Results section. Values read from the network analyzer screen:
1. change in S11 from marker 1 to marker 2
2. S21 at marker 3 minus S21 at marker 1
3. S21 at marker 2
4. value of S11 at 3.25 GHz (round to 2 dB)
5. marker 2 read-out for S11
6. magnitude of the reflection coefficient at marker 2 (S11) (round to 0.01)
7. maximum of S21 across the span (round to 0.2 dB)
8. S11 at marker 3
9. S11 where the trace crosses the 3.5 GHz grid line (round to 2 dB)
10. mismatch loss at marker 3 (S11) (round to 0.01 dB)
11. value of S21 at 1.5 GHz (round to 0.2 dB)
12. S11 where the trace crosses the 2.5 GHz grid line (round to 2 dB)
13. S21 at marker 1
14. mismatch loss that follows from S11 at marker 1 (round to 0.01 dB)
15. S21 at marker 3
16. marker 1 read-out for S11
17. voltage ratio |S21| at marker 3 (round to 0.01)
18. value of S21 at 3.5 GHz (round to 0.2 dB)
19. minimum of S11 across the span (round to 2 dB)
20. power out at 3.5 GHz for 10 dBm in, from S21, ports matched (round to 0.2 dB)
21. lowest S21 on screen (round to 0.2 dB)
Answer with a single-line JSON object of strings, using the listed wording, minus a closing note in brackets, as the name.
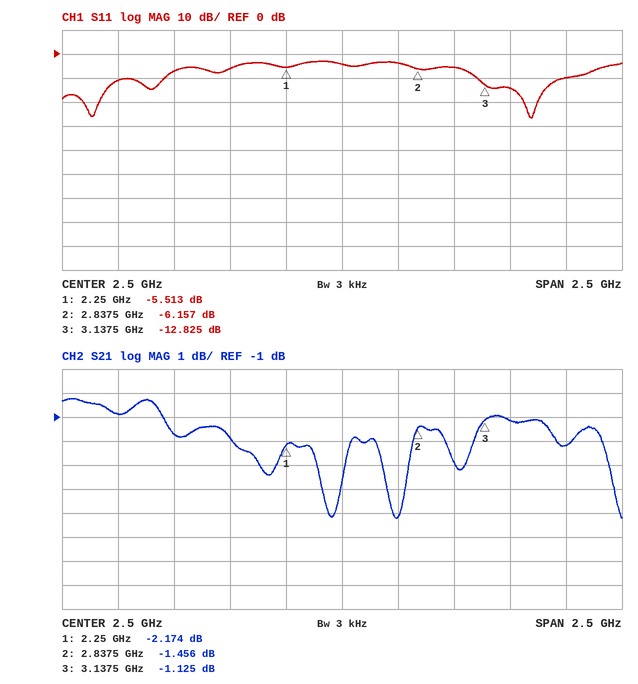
{"change in S11 from marker 1 to marker 2": "-0.644 dB", "S21 at marker 3 minus S21 at marker 1": "1.049 dB", "S21 at marker 2": "-1.456 dB", "value of S11 at 3.25 GHz": "-14 dB", "marker 2 read-out for S11": "-6.157 dB", "magnitude of the reflection coefficient at marker 2 (S11)": "0.49", "maximum of S21 across the span": "-0.2 dB", "S11 at marker 3": "-12.825 dB", "S11 where the trace crosses the 3.5 GHz grid line": "-10 dB", "mismatch loss at marker 3 (S11)": "0.23 dB", "value of S21 at 1.5 GHz": "-0.8 dB", "S11 where the trace crosses the 2.5 GHz grid line": "-4 dB", "S21 at marker 1": "-2.174 dB", "mismatch loss that follows from S11 at marker 1": "1.43 dB", "S21 at marker 3": "-1.125 dB", "marker 1 read-out for S11": "-5.513 dB", "voltage ratio |S21| at marker 3": "0.88", "value of S21 at 3.5 GHz": "-2.2 dB", "minimum of S11 across the span": "-26 dB", "power out at 3.5 GHz for 10 dBm in, from S21, ports matched": "7.8 dBm", "lowest S21 on screen": "-5.2 dB"}
